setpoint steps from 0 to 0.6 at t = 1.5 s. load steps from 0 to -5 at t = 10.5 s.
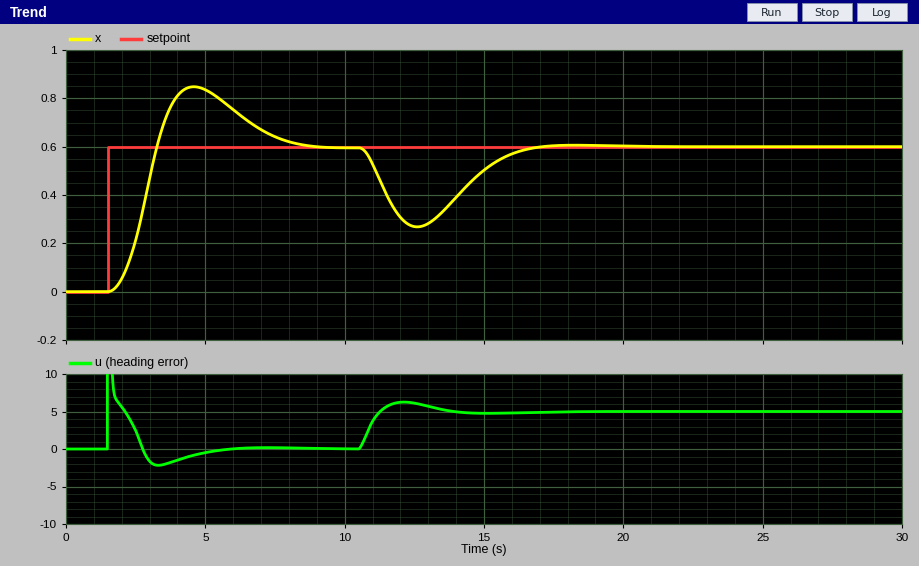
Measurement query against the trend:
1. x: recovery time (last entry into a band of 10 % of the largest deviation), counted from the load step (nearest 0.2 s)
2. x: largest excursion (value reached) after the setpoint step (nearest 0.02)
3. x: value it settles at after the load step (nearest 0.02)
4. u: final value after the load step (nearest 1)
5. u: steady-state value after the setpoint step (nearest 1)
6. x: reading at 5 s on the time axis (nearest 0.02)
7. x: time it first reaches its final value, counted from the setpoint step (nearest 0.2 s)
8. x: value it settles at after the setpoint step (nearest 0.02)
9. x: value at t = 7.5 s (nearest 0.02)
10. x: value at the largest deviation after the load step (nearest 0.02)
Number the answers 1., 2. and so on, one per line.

1. 5.4 s
2. 0.84
3. 0.60
4. 5
5. 0
6. 0.84
7. 1.8 s
8. 0.60
9. 0.64
10. 0.26
